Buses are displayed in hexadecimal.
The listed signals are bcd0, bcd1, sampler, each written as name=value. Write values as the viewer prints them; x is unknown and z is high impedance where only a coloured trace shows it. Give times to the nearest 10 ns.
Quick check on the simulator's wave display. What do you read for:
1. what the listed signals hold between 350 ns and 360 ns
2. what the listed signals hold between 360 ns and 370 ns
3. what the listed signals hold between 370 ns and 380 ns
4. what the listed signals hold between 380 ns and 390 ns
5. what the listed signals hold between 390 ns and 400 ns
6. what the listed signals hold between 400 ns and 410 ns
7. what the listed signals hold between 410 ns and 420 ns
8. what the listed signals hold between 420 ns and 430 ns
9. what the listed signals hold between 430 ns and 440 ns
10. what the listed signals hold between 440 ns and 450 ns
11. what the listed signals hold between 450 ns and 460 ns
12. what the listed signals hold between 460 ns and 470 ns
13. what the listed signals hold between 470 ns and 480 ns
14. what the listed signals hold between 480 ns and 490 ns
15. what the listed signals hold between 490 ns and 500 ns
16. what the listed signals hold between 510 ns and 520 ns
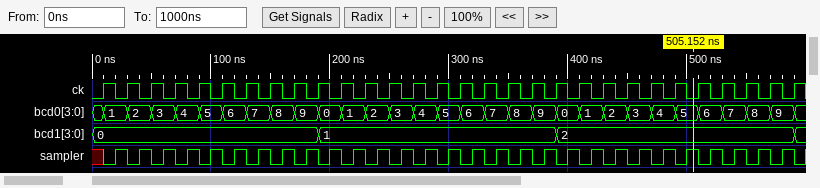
bcd0=8, bcd1=1, sampler=0
bcd0=8, bcd1=1, sampler=1
bcd0=9, bcd1=1, sampler=0
bcd0=9, bcd1=1, sampler=1
bcd0=0, bcd1=2, sampler=0
bcd0=0, bcd1=2, sampler=1
bcd0=1, bcd1=2, sampler=0
bcd0=1, bcd1=2, sampler=1
bcd0=2, bcd1=2, sampler=0
bcd0=2, bcd1=2, sampler=1
bcd0=3, bcd1=2, sampler=0
bcd0=3, bcd1=2, sampler=1
bcd0=4, bcd1=2, sampler=0
bcd0=4, bcd1=2, sampler=1
bcd0=5, bcd1=2, sampler=0
bcd0=6, bcd1=2, sampler=0
